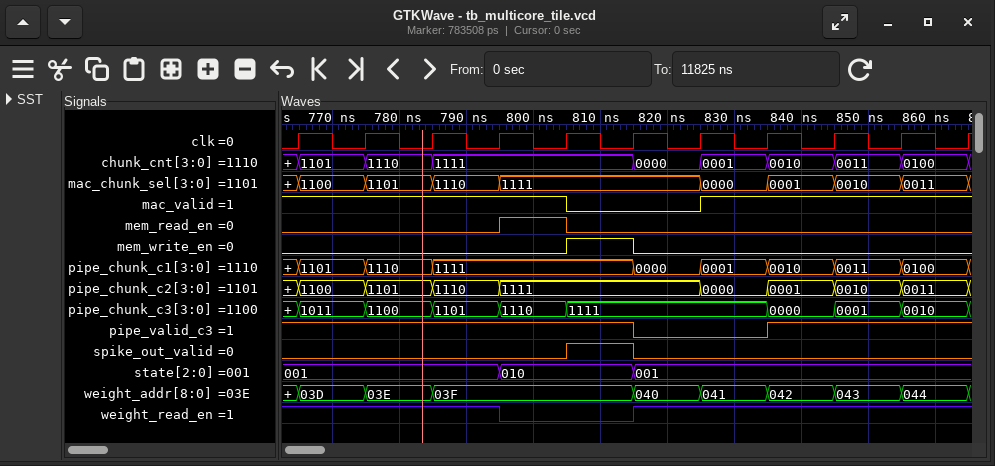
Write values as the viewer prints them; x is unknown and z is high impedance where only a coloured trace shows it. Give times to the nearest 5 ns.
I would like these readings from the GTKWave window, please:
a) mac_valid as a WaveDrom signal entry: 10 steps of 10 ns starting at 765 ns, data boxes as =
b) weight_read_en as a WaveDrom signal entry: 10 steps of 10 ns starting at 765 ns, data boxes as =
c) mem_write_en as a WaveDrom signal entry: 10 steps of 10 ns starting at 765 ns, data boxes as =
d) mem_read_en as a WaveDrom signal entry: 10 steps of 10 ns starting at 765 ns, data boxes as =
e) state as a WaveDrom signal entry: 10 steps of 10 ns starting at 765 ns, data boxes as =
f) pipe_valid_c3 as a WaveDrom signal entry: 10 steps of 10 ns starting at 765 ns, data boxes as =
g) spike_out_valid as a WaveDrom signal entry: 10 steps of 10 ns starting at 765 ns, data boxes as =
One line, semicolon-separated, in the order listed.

{name: 'mac_valid', wave: '1...0.1...'}; {name: 'weight_read_en', wave: '1..0.1....'}; {name: 'mem_write_en', wave: '0...10....'}; {name: 'mem_read_en', wave: '0..10.....'}; {name: 'state', wave: '=..=.=....', data: '001 010 001'}; {name: 'pipe_valid_c3', wave: '1....0.1..'}; {name: 'spike_out_valid', wave: '0...10....'}
